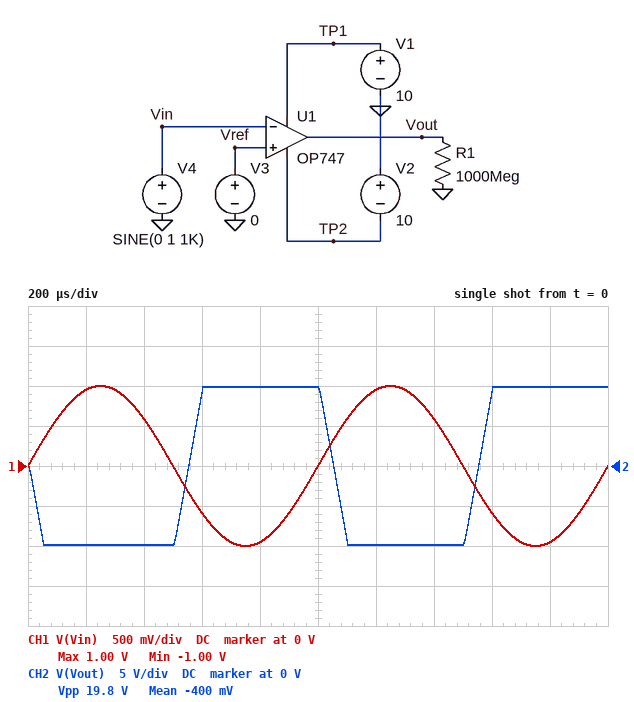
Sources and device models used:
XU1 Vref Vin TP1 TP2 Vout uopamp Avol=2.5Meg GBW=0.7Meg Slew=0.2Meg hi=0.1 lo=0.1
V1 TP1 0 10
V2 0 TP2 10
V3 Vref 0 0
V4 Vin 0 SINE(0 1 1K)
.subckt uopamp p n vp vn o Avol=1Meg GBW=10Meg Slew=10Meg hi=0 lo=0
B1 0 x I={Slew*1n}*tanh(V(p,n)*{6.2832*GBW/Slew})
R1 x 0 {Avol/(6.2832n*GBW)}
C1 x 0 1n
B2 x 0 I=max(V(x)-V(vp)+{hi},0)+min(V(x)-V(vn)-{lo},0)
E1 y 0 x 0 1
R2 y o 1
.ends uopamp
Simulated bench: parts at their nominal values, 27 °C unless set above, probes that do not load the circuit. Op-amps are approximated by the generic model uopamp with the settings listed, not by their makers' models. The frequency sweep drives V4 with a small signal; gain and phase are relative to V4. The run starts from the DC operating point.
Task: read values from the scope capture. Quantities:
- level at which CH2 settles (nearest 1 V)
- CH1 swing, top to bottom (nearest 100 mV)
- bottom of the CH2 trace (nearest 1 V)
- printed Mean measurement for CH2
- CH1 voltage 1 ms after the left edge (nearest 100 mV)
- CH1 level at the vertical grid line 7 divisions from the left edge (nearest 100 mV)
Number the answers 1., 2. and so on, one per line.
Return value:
1. 10 V
2. 2.0 V
3. -10 V
4. -400 mV
5. 0 V
6. 600 mV
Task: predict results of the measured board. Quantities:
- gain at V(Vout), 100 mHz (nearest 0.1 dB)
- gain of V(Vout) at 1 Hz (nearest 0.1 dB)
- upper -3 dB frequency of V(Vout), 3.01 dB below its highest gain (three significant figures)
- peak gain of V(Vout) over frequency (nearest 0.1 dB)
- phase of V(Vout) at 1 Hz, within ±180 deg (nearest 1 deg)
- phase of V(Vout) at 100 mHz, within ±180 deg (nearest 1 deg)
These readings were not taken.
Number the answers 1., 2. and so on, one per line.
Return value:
1. 127.4 dB
2. 116.6 dB
3. 280 mHz
4. 128.0 dB
5. 106 deg
6. 160 deg
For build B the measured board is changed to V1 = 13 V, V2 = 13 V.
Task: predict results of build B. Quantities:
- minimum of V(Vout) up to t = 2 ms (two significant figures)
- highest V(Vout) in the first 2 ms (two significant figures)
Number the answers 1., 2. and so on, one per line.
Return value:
1. -13 V
2. 13 V
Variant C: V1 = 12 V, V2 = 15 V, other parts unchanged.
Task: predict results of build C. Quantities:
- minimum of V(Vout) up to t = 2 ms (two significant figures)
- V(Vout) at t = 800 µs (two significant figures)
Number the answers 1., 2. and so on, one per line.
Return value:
1. -15 V
2. 12 V
